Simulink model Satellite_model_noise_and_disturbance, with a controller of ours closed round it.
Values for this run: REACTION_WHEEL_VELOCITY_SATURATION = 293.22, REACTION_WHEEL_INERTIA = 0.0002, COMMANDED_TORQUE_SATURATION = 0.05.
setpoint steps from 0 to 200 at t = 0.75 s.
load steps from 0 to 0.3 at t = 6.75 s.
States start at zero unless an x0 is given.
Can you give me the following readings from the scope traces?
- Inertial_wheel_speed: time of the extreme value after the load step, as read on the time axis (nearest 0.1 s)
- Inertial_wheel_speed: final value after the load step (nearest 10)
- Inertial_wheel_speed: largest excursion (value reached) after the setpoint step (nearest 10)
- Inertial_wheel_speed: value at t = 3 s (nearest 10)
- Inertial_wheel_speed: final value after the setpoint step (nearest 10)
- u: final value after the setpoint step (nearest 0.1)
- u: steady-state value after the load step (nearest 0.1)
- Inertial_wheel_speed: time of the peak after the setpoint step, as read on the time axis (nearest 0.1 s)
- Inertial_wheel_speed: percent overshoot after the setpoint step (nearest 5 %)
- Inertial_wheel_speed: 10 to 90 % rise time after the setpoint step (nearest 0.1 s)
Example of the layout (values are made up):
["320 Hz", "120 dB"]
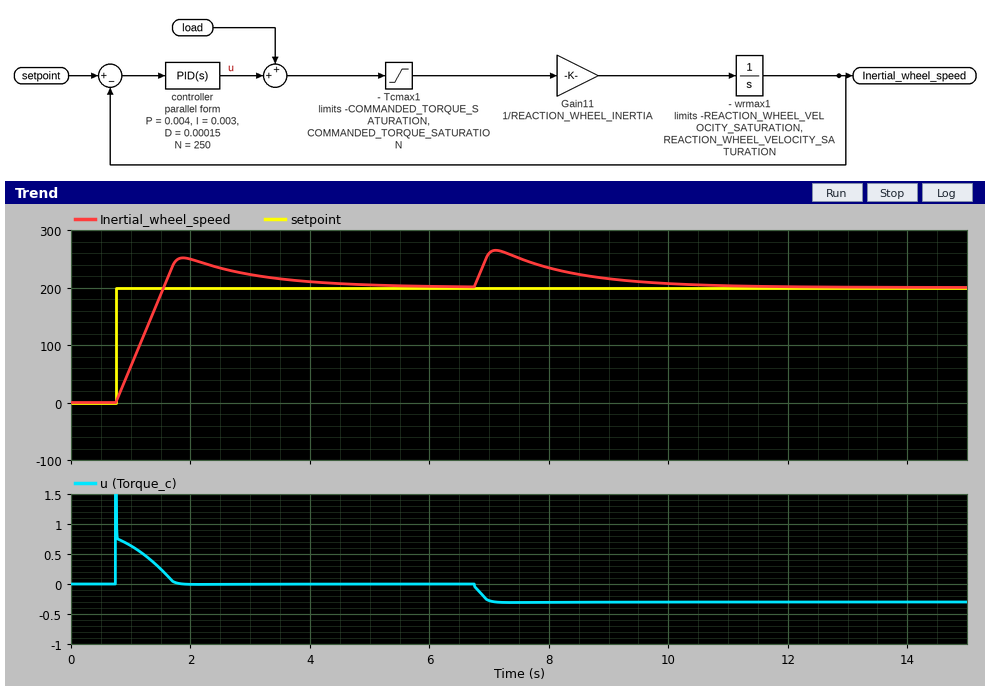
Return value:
["7.1 s", "200", "250", "220", "200", "0.0", "-0.3", "1.9 s", "25 %", "0.6 s"]
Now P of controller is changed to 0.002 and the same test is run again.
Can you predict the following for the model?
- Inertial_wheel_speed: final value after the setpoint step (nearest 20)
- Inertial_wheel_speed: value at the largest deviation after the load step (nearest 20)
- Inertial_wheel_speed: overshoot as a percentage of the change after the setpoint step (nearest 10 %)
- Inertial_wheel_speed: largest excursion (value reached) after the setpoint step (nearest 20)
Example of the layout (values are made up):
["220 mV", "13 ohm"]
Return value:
["200", "300", "40 %", "280"]
